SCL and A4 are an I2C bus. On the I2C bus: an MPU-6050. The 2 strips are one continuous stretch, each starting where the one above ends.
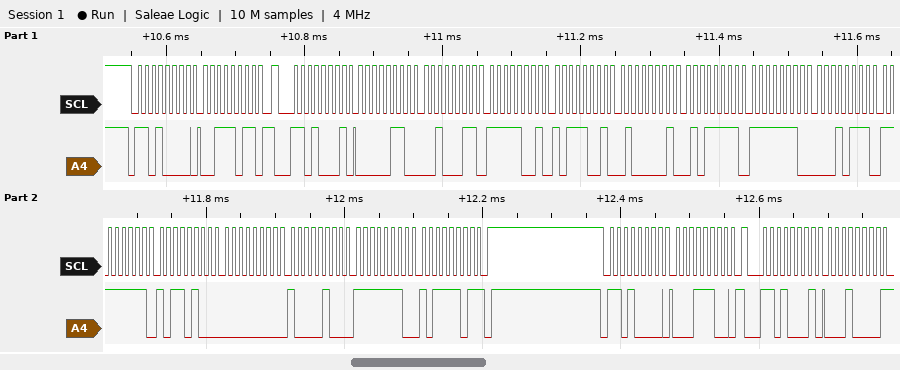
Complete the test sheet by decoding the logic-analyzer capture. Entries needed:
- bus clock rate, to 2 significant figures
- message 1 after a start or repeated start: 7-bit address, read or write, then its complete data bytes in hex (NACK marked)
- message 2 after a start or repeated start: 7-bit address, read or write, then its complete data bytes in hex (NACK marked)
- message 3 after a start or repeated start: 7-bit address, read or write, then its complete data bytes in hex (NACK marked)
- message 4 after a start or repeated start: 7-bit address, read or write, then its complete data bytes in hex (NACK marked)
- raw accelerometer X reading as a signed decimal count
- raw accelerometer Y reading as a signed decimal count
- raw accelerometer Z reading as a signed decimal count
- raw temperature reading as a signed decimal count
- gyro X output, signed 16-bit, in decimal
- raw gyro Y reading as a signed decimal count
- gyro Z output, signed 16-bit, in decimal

100 kHz
0x68 write: 3B
0x68 read: 06 23 F9 B9 41 5F FE 17 FF B4 00 84 FE BD NACK
0x68 write: 1C
0x68 read: 10 NACK
1571
-1607
16735
-489
-76
132
-323
